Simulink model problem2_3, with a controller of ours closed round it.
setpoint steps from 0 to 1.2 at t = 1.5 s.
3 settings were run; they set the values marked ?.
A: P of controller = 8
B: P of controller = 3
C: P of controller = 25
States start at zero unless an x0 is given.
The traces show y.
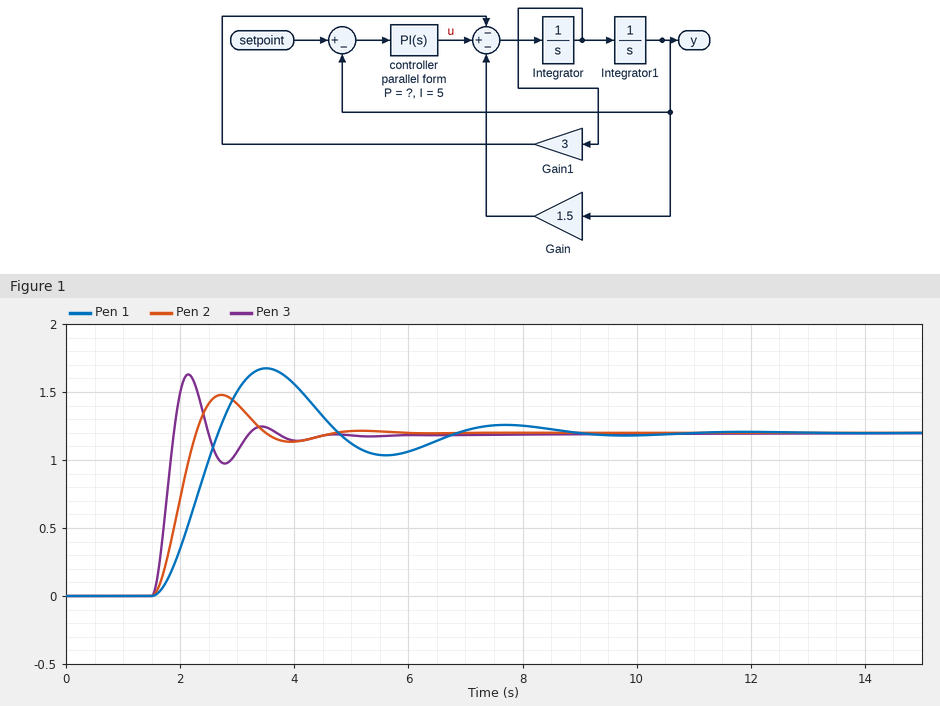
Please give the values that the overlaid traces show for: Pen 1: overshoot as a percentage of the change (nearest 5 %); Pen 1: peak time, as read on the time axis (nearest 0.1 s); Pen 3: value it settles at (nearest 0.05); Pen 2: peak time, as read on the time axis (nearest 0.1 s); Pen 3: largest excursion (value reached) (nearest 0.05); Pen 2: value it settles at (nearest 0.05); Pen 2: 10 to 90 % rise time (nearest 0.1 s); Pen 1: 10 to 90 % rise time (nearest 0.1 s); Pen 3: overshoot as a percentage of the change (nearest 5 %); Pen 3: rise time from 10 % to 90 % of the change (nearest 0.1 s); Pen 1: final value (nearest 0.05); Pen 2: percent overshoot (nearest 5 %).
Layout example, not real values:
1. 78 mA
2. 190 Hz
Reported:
1. 40 %
2. 3.5 s
3. 1.20
4. 2.7 s
5. 1.65
6. 1.20
7. 0.5 s
8. 0.8 s
9. 35 %
10. 0.3 s
11. 1.20
12. 25 %
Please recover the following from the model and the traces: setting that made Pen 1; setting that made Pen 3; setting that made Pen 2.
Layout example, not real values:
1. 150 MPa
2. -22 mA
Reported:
1. B
2. C
3. A
